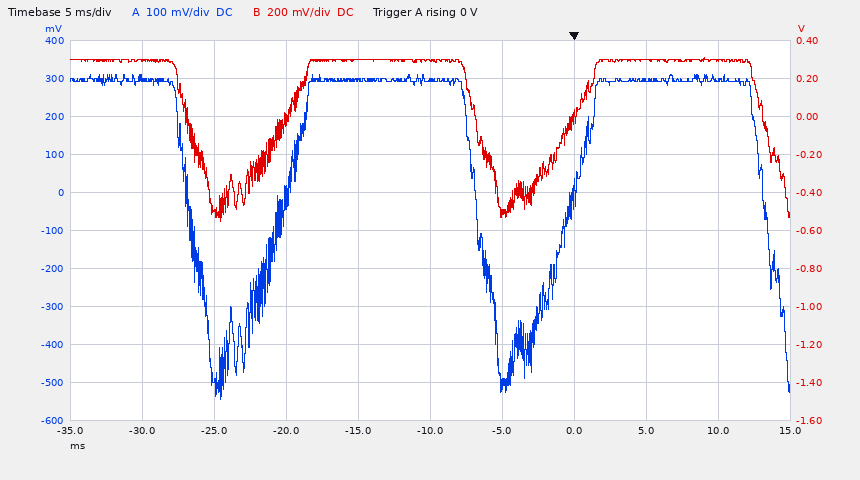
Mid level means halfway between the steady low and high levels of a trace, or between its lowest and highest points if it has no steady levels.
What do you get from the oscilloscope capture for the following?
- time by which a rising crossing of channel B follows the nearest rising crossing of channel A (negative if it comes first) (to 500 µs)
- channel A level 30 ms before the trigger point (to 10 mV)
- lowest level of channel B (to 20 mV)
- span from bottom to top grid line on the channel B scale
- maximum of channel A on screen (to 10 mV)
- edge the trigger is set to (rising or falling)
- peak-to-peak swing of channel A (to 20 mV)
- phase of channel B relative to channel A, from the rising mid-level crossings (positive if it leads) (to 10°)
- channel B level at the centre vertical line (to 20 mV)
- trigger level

0.0 ms
300 mV
-560 mV
2 V
310 mV
rising
860 mV
0°
300 mV
0 V
